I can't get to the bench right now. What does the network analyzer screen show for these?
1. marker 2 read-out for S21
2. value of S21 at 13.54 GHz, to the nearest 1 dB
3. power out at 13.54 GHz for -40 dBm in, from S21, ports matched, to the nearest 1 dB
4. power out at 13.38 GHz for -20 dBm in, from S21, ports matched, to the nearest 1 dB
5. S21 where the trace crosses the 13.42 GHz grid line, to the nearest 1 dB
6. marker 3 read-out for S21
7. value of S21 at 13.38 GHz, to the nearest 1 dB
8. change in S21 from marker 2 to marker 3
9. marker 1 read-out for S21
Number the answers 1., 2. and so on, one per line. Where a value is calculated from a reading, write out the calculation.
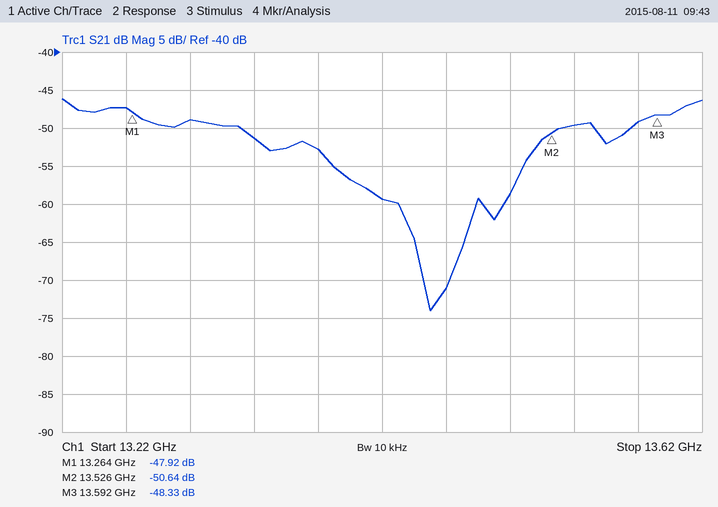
1. -50.64 dB
2. -50 dB
3. -40 dBm + (-50 dB) = -90 dBm
4. -20 dBm + (-53 dB) = -73 dBm
5. -59 dB
6. -48.33 dB
7. -53 dB
8. -48.33 − (-50.64) = 2.31 dB
9. -47.92 dB
